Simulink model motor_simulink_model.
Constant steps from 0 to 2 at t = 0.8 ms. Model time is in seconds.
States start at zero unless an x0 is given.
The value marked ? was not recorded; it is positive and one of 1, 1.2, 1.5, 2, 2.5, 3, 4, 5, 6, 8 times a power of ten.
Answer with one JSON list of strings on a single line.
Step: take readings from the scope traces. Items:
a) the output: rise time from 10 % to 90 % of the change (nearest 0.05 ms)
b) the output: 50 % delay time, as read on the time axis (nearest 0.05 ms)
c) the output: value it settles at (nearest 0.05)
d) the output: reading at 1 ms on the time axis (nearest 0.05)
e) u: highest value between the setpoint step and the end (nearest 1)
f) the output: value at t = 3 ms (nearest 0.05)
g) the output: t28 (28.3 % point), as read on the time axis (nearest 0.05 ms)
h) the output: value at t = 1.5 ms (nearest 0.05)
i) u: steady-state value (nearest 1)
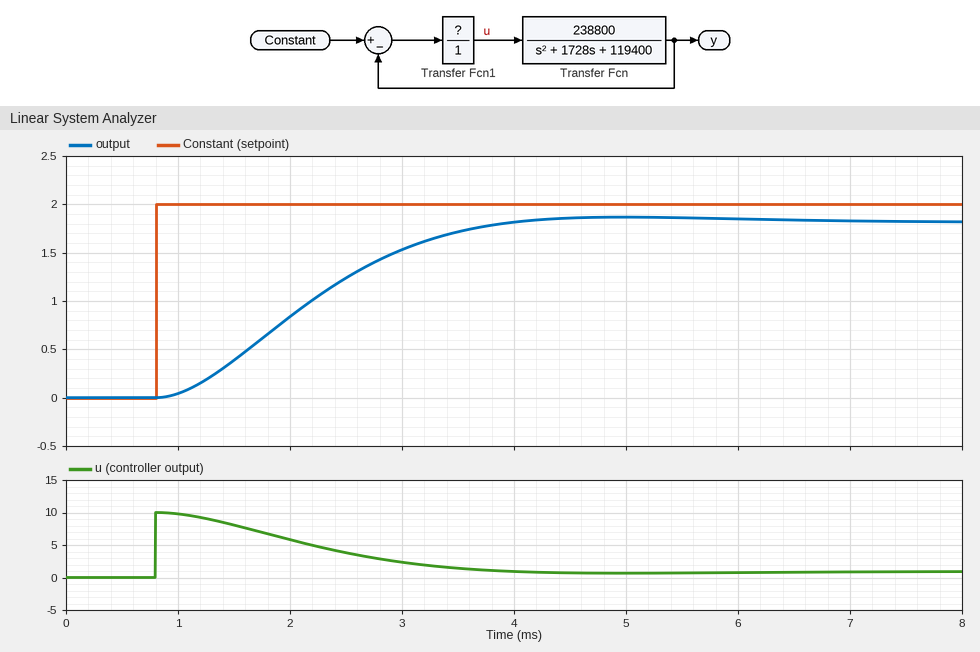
["2.00 ms", "2.10 ms", "1.80", "0.05", "10", "1.55", "1.65 ms", "0.40", "1"]
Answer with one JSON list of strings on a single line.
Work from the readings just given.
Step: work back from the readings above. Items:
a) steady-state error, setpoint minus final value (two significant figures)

["0.20"]
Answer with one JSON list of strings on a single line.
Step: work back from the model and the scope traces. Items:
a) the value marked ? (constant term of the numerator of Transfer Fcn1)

["5"]
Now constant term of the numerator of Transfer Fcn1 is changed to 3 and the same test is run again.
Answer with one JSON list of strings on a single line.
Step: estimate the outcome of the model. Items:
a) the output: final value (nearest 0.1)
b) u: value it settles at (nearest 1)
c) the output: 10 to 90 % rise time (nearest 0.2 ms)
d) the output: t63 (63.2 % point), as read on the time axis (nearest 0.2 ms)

["1.7", "1", "3.4 ms", "3.0 ms"]
